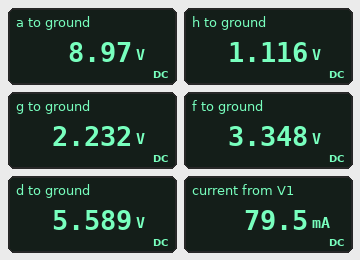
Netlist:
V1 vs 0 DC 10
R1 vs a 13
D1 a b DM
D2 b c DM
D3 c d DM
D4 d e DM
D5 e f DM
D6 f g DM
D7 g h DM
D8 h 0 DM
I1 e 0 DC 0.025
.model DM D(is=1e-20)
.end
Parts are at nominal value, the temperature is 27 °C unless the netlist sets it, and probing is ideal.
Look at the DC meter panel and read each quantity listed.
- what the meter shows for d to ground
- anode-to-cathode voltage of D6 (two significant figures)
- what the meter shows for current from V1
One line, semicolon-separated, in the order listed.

5.589 V; 1.1 V; 79.5 mA
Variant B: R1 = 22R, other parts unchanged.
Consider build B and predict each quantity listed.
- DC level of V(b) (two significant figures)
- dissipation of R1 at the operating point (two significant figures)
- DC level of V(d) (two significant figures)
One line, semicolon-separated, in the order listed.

7.7 V; 60 mW; 5.5 V
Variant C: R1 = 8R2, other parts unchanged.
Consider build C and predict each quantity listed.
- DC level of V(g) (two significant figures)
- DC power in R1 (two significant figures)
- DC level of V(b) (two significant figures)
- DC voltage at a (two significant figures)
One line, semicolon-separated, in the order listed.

2.3 V; 110 mW; 7.9 V; 9.1 V
